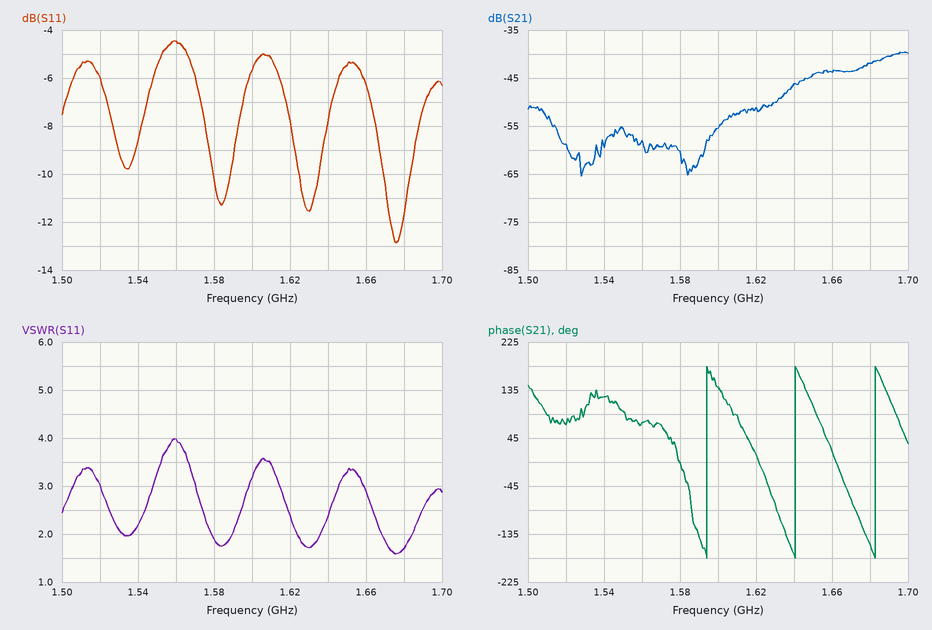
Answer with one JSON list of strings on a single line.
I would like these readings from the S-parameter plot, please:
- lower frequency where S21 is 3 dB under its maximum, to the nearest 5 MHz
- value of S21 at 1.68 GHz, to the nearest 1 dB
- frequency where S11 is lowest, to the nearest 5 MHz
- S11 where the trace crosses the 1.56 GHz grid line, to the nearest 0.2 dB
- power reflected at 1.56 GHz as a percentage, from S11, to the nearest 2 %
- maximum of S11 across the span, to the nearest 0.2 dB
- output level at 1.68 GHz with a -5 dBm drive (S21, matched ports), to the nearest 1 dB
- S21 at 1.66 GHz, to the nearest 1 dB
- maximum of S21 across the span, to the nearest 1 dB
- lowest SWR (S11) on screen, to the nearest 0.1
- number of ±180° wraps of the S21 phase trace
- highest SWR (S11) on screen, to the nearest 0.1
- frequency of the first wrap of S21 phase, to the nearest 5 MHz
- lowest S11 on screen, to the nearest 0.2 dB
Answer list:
["1.675 GHz", "-42 dB", "1.675 GHz", "-4.4 dB", "36 %", "-4.4 dB", "-47 dBm", "-44 dB", "-40 dB", "1.6", "3", "4.0", "1.595 GHz", "-12.8 dB"]
